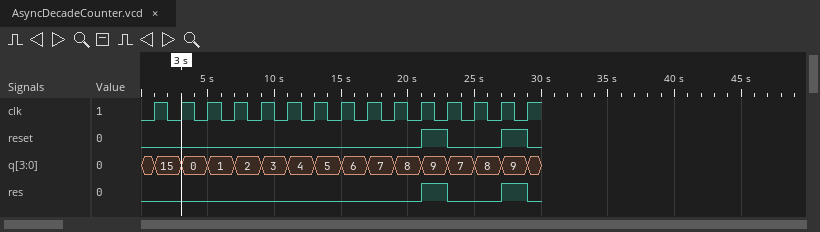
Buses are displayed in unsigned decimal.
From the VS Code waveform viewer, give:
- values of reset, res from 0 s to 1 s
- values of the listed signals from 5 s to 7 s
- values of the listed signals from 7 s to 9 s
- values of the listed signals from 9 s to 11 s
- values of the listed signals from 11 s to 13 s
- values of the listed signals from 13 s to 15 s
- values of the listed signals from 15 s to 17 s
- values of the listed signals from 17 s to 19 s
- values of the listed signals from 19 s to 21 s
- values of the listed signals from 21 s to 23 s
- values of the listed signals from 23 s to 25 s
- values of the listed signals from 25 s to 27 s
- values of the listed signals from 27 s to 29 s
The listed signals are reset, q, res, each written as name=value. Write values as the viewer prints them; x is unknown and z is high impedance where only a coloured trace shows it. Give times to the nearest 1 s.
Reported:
reset=0, res=0
reset=0, q=1, res=0
reset=0, q=2, res=0
reset=0, q=3, res=0
reset=0, q=4, res=0
reset=0, q=5, res=0
reset=0, q=6, res=0
reset=0, q=7, res=0
reset=0, q=8, res=0
reset=1, q=9, res=1
reset=0, q=7, res=0
reset=0, q=8, res=0
reset=1, q=9, res=1
